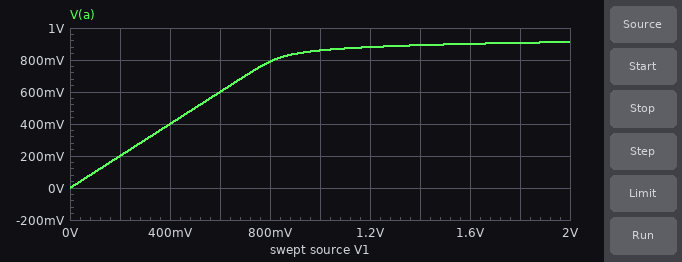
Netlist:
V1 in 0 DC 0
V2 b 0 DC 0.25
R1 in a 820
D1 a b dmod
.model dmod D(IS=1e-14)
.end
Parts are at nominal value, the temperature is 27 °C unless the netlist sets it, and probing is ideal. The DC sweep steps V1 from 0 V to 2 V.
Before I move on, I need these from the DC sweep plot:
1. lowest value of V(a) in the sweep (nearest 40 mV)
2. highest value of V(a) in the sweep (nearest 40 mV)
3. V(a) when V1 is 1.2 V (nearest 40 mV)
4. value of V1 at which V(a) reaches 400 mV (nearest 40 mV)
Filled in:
0 V
920 mV
880 mV
400 mV
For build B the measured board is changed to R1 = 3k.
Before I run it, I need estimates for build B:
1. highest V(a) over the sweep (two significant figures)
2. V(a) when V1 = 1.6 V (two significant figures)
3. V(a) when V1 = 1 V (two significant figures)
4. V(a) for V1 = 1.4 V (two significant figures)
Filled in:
880 mV
870 mV
830 mV
860 mV
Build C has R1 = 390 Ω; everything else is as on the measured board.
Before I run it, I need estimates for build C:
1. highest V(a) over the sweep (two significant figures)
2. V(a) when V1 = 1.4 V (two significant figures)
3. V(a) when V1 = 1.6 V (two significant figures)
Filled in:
930 mV
910 mV
920 mV
